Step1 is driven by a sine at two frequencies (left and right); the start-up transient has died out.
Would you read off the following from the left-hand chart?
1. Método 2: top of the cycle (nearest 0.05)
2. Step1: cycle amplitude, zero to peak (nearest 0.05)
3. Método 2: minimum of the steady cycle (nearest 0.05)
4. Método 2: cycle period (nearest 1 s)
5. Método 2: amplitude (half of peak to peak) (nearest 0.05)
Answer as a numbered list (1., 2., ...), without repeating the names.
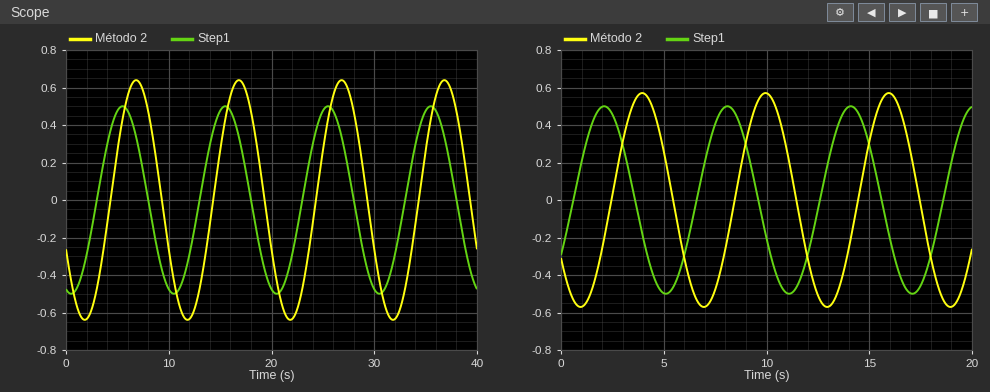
1. 0.65
2. 0.50
3. -0.65
4. 10 s
5. 0.65
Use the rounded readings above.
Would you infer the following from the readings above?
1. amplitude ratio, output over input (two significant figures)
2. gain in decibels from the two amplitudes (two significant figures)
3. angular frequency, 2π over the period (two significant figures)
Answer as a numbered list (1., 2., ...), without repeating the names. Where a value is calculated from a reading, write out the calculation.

1. 0.65 / 0.5 = 1.3
2. 20 log10(0.65 / 0.5) = 2.3 dB
3. 2π / 10 = 0.63 rad/s
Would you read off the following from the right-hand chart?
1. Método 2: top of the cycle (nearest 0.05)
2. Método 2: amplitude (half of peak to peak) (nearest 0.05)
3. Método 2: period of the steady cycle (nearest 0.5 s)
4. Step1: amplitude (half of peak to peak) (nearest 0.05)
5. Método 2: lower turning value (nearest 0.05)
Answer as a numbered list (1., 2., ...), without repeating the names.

1. 0.55
2. 0.55
3. 6.0 s
4. 0.50
5. -0.55
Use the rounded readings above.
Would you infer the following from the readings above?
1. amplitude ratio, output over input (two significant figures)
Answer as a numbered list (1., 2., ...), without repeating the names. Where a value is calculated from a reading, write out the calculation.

1. 0.55 / 0.5 = 1.1
